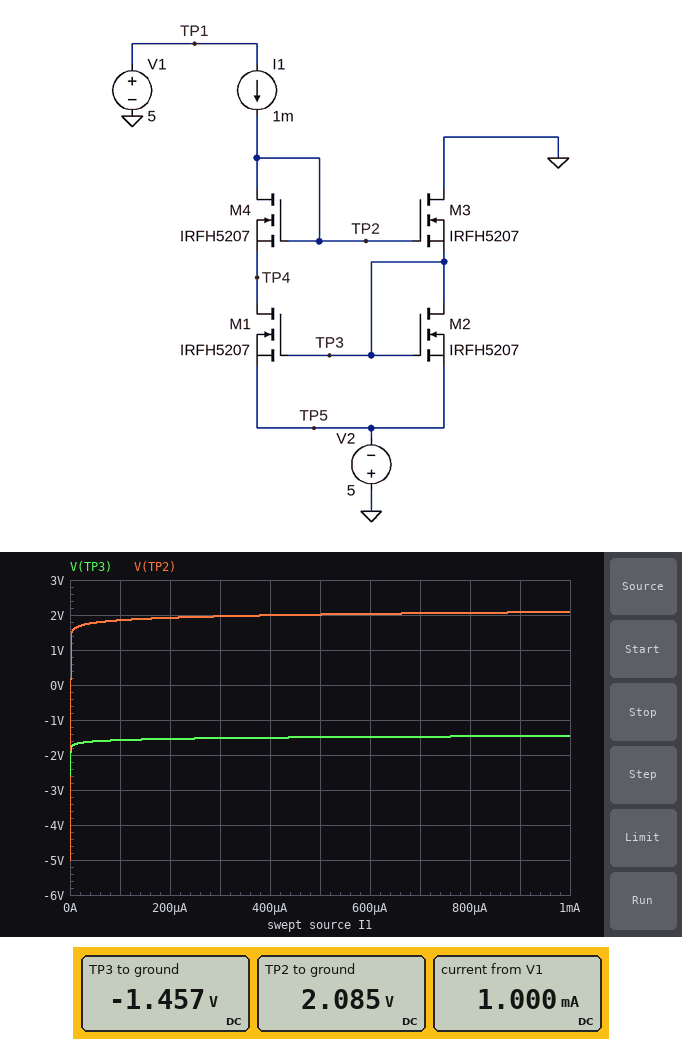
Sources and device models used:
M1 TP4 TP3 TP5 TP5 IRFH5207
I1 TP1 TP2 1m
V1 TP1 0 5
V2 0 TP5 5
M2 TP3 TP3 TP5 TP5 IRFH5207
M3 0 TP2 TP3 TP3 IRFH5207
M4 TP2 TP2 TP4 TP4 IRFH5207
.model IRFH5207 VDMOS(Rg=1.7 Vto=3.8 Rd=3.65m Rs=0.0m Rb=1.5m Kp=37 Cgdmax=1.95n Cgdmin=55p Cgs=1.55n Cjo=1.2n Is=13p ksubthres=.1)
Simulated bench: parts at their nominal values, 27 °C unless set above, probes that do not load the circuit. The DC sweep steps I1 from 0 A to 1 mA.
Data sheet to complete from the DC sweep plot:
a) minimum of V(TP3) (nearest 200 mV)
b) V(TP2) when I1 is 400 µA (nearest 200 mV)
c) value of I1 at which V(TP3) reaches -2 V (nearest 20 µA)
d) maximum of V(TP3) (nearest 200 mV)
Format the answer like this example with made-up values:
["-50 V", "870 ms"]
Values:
["-2.6 V", "2.0 V", "0 A", "-1.4 V"]
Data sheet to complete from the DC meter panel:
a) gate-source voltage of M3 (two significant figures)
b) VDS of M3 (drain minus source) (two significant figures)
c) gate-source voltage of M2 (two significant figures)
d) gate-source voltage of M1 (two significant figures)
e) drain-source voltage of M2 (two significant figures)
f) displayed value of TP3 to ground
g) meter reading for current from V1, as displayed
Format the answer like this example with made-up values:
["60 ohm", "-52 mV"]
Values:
["3.5 V", "1.5 V", "3.5 V", "3.5 V", "3.5 V", "-1.457 V", "1.000 mA"]
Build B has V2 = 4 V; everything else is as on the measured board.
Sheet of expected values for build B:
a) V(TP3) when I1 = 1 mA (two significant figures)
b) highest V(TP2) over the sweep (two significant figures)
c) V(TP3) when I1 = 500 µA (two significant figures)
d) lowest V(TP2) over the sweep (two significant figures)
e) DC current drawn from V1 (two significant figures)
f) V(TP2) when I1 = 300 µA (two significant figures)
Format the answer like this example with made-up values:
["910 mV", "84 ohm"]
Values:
["-460 mV", "3.1 V", "-490 mV", "-4.0 V", "1.0 mA", "3.0 V"]
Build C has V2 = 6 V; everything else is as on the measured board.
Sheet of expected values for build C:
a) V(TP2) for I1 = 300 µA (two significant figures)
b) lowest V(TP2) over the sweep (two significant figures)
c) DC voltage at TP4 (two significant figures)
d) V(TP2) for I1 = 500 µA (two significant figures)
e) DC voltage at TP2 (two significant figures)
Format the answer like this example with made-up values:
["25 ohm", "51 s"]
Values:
["960 mV", "-6.0 V", "-2.5 V", "1.0 V", "1.1 V"]
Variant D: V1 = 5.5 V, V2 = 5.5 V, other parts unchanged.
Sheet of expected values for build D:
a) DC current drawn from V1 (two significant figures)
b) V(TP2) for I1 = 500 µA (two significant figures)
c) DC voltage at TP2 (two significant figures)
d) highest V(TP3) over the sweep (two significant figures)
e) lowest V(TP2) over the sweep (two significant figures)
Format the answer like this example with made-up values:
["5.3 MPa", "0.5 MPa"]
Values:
["1.0 mA", "1.5 V", "1.6 V", "-2.0 V", "-5.5 V"]
